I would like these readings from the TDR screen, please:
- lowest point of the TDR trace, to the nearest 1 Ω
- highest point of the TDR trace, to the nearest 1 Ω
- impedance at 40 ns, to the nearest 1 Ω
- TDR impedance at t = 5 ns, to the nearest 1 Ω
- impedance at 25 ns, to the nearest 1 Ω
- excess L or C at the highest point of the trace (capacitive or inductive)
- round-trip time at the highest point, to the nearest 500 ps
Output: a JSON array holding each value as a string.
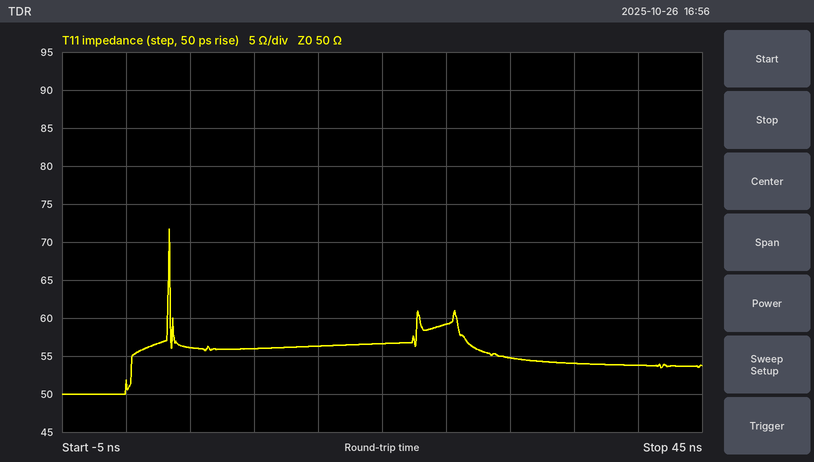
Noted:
["50 Ω", "72 Ω", "54 Ω", "56 Ω", "59 Ω", "inductive", "3.5 ns"]
